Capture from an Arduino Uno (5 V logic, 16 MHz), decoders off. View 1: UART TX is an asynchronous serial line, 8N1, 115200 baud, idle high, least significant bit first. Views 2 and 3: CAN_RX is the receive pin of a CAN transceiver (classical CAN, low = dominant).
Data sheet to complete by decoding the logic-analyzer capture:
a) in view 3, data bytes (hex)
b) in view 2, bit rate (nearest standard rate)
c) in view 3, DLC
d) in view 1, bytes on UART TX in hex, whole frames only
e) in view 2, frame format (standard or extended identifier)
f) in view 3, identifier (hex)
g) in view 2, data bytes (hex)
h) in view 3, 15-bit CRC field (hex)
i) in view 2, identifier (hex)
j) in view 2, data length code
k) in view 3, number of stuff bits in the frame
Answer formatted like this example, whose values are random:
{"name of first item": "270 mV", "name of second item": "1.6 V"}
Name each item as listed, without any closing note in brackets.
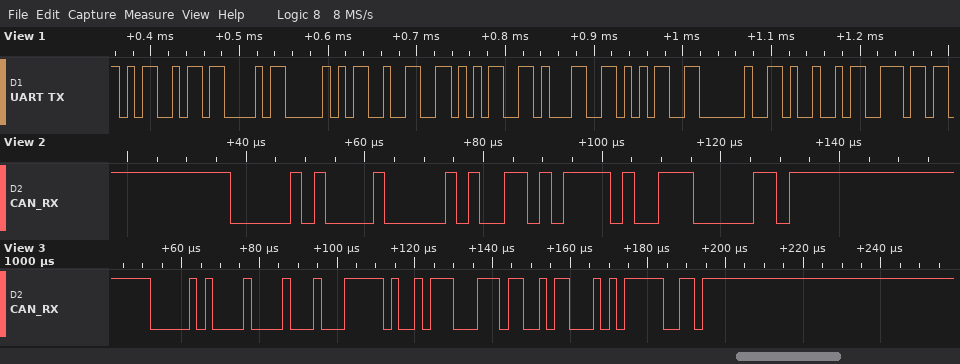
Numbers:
{"in view 3, data bytes": "47 E5 C7 65", "in view 2, bit rate": "500 kbit/s", "in view 3, DLC": "4", "in view 1, bytes on UART TX in hex, whole frames only": "4D 43 50 32 35 31 35 20 49 6E", "in view 2, frame format": "standard", "in view 3, identifier": "0x021", "in view 2, data bytes": "35", "in view 3, 15-bit CRC field": "0x457D", "in view 2, identifier": "0x021", "in view 2, data length code": "1", "in view 3, number of stuff bits in the frame": "3"}
